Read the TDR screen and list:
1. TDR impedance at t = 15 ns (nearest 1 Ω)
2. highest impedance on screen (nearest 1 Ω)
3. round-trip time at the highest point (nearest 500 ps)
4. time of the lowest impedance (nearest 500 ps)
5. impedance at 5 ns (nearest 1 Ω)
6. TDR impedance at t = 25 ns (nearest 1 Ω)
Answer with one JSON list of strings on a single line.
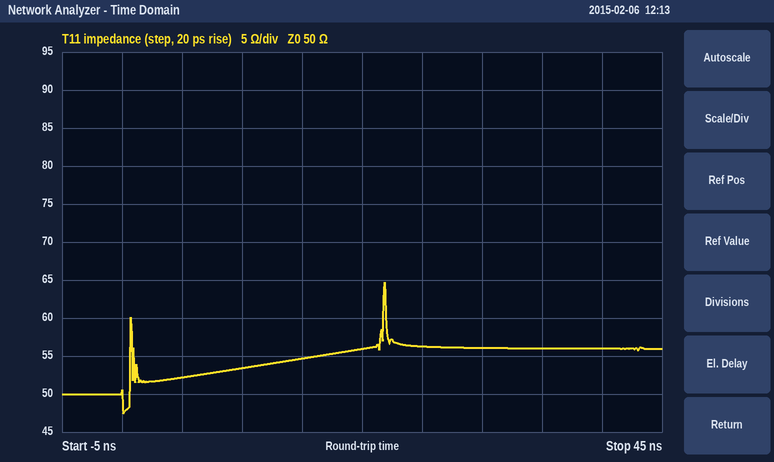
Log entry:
["55 Ω", "65 Ω", "22.0 ns", "0.0 ns", "52 Ω", "56 Ω"]
